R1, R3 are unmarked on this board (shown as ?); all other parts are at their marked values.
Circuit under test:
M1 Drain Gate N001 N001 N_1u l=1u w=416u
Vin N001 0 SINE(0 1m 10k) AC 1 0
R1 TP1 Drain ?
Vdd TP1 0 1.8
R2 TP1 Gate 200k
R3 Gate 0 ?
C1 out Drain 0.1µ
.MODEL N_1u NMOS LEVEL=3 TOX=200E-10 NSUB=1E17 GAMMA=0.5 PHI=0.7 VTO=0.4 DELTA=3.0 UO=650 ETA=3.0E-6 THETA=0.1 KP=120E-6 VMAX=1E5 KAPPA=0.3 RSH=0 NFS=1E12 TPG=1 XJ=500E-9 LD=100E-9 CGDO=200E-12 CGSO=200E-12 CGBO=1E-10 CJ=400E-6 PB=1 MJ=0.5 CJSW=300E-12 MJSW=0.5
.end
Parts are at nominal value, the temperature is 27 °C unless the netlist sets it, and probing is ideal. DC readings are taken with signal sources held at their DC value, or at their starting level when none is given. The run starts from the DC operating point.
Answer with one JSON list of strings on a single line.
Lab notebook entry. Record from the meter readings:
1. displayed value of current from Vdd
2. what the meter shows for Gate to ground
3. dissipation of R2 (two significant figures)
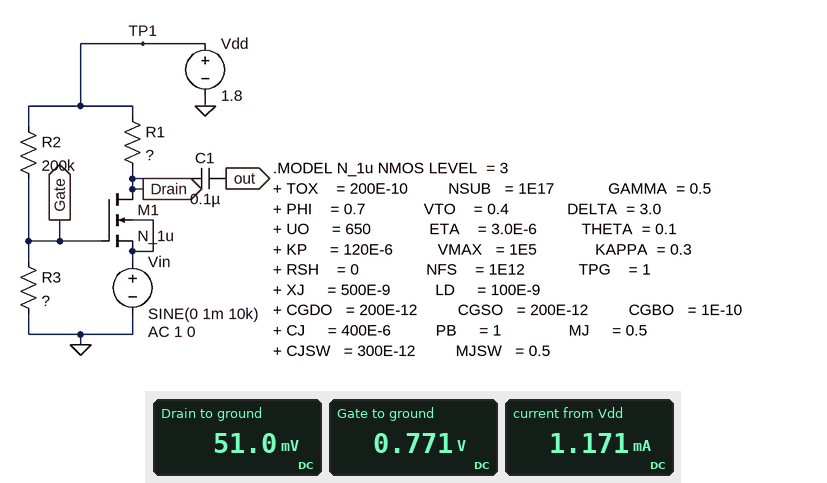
["1.171 mA", "0.771 V", "5.3 µW"]
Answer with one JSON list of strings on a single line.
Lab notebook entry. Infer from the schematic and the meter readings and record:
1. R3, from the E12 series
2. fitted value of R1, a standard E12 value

["150 kΩ", "1.5 kΩ"]
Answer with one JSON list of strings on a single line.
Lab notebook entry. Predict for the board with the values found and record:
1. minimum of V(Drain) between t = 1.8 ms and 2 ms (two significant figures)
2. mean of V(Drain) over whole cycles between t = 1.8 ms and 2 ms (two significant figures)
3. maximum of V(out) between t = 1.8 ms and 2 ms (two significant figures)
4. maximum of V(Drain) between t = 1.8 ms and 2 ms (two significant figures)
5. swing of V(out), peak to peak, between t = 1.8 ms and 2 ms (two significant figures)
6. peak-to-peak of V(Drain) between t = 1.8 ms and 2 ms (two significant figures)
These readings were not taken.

["50 mV", "51 mV", "1.1 mV", "52 mV", "2.2 mV", "2.2 mV"]
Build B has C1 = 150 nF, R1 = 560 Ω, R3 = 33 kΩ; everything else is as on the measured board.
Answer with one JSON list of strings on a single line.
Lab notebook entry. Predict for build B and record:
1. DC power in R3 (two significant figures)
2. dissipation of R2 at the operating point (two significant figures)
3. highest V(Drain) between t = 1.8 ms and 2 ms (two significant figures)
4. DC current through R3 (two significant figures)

["2.0 µW", "12 µW", "1.8 V", "7.7 µA"]
